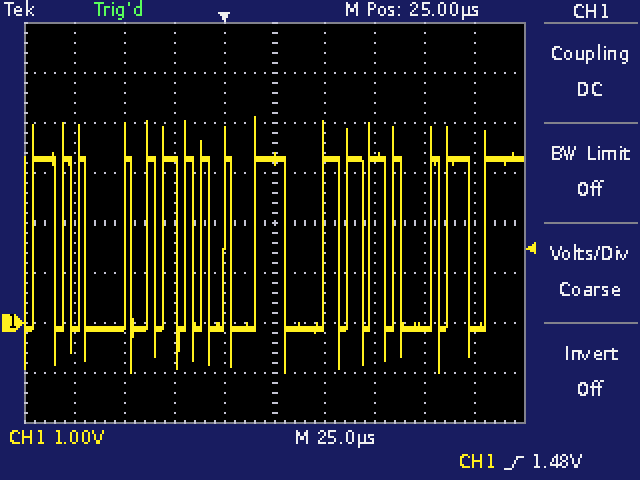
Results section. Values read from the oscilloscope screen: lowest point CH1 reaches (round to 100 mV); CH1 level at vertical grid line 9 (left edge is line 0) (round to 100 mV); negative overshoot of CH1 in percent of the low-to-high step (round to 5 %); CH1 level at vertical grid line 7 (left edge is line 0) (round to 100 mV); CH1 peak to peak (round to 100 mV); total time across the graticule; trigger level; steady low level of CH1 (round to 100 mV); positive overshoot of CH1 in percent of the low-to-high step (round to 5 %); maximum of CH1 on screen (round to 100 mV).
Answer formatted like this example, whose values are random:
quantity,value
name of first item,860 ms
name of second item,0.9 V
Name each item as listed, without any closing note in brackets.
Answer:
quantity,value
lowest point CH1 reaches,-1.0 V
CH1 level at vertical grid line 9 (left edge is line 0),-100 mV
negative overshoot of CH1 in percent of the low-to-high step,25 %
CH1 level at vertical grid line 7 (left edge is line 0),3.3 V
CH1 peak to peak,5.1 V
total time across the graticule,250 µs
trigger level,1.48 V
steady low level of CH1,-100 mV
positive overshoot of CH1 in percent of the low-to-high step,25 %
maximum of CH1 on screen,4.1 V
